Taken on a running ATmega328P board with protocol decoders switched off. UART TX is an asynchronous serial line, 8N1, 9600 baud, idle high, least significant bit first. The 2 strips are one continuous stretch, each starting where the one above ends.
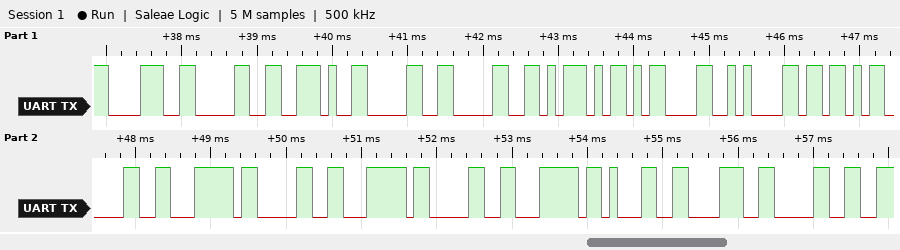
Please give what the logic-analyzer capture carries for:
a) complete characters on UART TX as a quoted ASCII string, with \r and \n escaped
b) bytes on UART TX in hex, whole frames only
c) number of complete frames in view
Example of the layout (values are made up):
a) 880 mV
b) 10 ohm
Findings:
a) "80.00]\r\n[0|0|0|180"
b) 0x38 0x30 0x2E 0x30 0x30 0x5D 0x0D 0x0A 0x5B 0x30 0x7C 0x30 0x7C 0x30 0x7C 0x31 0x38 0x30
c) 18
